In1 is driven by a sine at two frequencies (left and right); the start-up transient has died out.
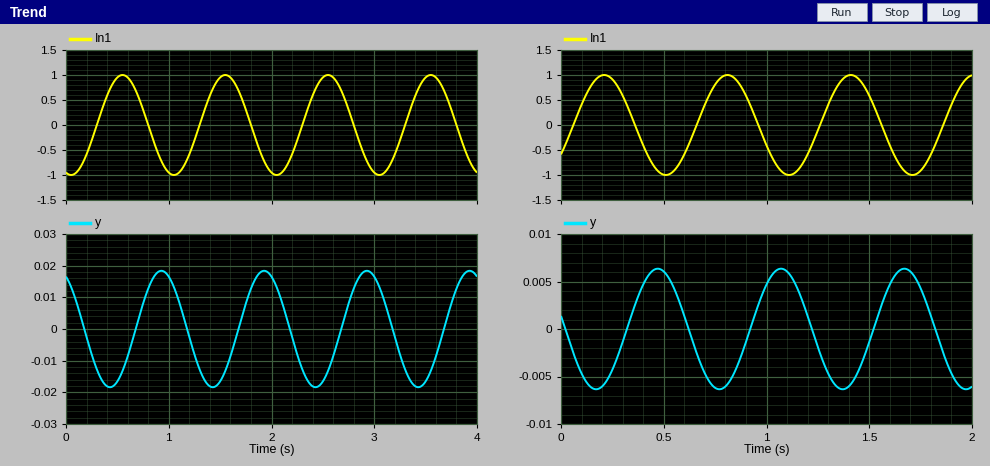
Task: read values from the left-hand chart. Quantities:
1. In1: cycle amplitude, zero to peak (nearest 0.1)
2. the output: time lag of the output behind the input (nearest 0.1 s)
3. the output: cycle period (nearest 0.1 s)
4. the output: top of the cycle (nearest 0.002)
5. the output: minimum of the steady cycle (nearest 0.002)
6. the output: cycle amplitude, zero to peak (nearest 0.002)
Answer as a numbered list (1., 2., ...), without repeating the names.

1. 1.0
2. 0.4 s
3. 1.0 s
4. 0.018
5. -0.018
6. 0.018
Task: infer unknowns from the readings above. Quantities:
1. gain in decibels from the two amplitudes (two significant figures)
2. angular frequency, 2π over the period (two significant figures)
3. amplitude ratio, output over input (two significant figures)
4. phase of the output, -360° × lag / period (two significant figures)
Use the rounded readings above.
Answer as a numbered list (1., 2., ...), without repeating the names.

1. -35 dB
2. 6.3 rad/s
3. 0.018
4. -140°
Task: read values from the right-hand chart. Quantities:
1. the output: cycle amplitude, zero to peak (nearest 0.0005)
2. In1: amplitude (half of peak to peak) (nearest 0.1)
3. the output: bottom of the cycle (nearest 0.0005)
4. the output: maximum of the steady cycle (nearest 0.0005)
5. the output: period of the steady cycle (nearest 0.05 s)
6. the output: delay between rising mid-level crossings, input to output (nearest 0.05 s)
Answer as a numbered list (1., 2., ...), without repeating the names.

1. 0.0065
2. 1.0
3. -0.0065
4. 0.0065
5. 0.60 s
6. 0.25 s
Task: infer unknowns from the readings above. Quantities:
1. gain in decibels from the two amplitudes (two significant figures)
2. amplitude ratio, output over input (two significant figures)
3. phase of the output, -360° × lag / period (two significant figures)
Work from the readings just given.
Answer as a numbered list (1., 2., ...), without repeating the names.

1. -44 dB
2. 0.0065
3. -150°
